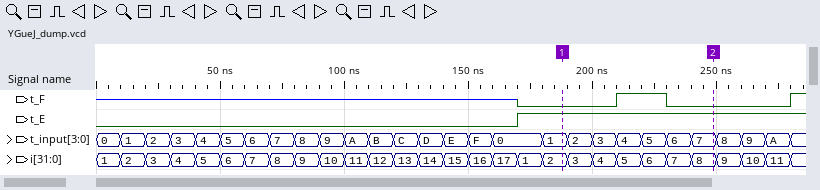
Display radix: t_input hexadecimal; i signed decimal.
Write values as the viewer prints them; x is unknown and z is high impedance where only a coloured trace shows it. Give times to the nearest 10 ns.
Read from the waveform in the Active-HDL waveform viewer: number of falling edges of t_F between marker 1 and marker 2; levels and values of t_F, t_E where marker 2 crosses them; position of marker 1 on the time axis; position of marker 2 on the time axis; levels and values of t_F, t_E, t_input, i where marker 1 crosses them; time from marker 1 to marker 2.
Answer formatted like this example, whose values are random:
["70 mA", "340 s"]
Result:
["1", "t_F=0, t_E=1", "190 ns", "250 ns", "t_F=0, t_E=1, t_input=1, i=2", "60 ns"]
